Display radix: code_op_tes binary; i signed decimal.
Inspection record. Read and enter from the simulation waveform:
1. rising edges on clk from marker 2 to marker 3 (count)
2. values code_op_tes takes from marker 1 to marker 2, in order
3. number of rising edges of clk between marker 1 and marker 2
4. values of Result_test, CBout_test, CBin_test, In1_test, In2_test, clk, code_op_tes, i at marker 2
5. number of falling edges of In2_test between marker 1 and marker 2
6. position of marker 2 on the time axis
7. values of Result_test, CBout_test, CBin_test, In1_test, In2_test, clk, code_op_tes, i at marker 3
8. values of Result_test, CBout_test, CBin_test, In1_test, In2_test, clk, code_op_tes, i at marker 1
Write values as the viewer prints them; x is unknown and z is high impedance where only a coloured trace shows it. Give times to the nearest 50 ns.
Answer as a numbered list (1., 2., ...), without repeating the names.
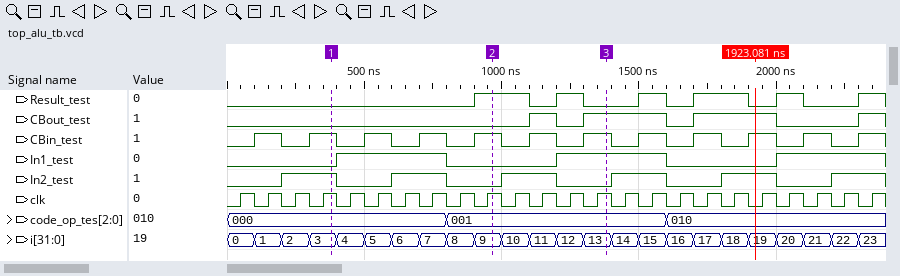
1. 4
2. 000, 001
3. 6
4. Result_test=1, CBout_test=0, CBin_test=1, In1_test=0, In2_test=0, clk=1, code_op_tes=001, i=9
5. 2
6. 950 ns
7. Result_test=0, CBout_test=1, CBin_test=1, In1_test=1, In2_test=0, clk=1, code_op_tes=001, i=13
8. Result_test=0, CBout_test=0, CBin_test=1, In1_test=0, In2_test=1, clk=1, code_op_tes=000, i=3
